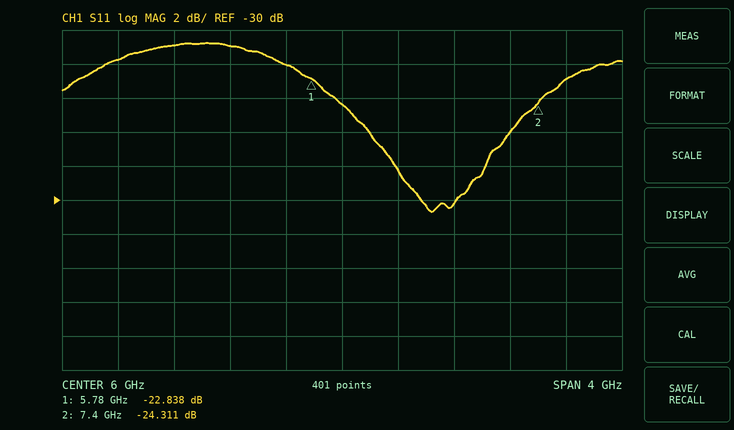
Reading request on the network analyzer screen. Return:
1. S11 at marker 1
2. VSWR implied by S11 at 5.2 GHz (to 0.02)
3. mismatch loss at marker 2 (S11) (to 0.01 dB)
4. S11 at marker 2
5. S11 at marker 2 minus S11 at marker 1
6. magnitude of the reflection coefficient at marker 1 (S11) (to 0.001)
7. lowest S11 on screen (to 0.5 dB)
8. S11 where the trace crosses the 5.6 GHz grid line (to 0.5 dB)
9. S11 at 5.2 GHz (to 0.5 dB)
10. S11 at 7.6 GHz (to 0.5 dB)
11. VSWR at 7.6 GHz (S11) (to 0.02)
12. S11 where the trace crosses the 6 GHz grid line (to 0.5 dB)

-22.838 dB
1.20
0.02 dB
-24.311 dB
-1.473 dB
0.072
-30.5 dB
-22.0 dB
-21.0 dB
-23.0 dB
1.16
-24.5 dB
